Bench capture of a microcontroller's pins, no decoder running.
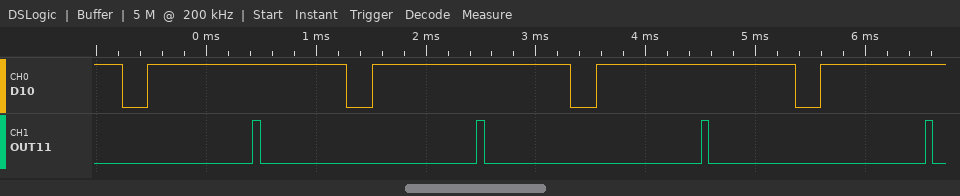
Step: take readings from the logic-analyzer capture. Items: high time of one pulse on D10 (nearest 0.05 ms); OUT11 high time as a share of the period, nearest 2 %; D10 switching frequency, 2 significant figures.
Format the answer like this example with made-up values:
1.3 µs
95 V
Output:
1.80 ms
4 %
490 Hz
